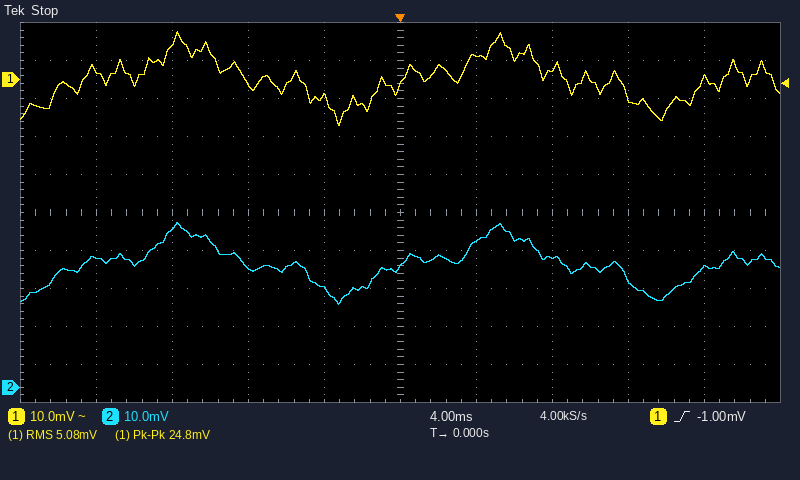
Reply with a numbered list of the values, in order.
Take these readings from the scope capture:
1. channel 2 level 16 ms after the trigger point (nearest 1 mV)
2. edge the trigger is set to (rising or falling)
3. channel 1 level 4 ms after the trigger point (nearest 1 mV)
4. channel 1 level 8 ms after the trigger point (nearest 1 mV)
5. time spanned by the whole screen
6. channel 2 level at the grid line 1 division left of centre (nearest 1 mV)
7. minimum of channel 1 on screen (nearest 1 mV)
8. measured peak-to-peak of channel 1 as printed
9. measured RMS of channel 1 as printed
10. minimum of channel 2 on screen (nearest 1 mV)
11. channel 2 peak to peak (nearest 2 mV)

1. 31 mV
2. rising
3. 6 mV
4. 3 mV
5. 40 ms
6. 26 mV
7. -12 mV
8. 24.8 mV
9. 5.08 mV
10. 22 mV
11. 22 mV
